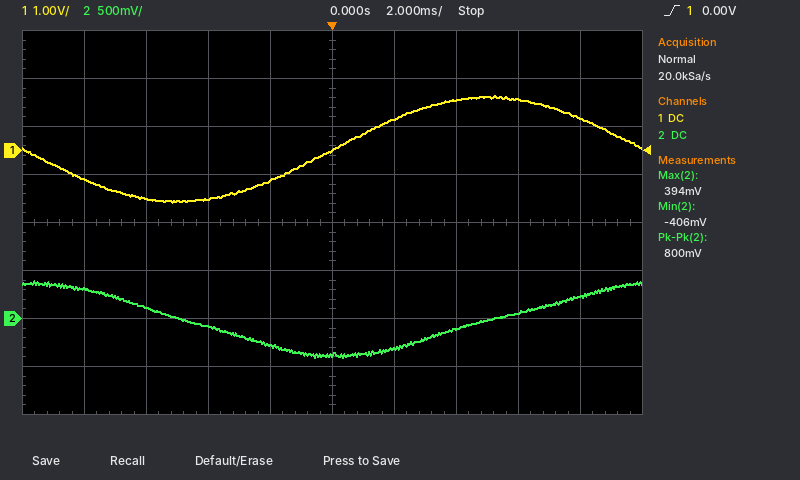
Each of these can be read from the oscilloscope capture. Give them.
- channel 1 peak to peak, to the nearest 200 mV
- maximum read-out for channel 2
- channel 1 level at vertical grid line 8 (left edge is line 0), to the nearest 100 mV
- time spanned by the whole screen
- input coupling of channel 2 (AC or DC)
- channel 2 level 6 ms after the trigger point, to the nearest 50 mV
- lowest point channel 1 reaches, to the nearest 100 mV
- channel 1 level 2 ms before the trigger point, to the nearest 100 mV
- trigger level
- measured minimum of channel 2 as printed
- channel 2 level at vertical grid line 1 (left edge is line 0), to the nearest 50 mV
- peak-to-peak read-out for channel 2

2.2 V
394 mV
1.1 V
20 ms
DC
50 mV
-1.1 V
-600 mV
0.00 V
-406 mV
300 mV
800 mV
